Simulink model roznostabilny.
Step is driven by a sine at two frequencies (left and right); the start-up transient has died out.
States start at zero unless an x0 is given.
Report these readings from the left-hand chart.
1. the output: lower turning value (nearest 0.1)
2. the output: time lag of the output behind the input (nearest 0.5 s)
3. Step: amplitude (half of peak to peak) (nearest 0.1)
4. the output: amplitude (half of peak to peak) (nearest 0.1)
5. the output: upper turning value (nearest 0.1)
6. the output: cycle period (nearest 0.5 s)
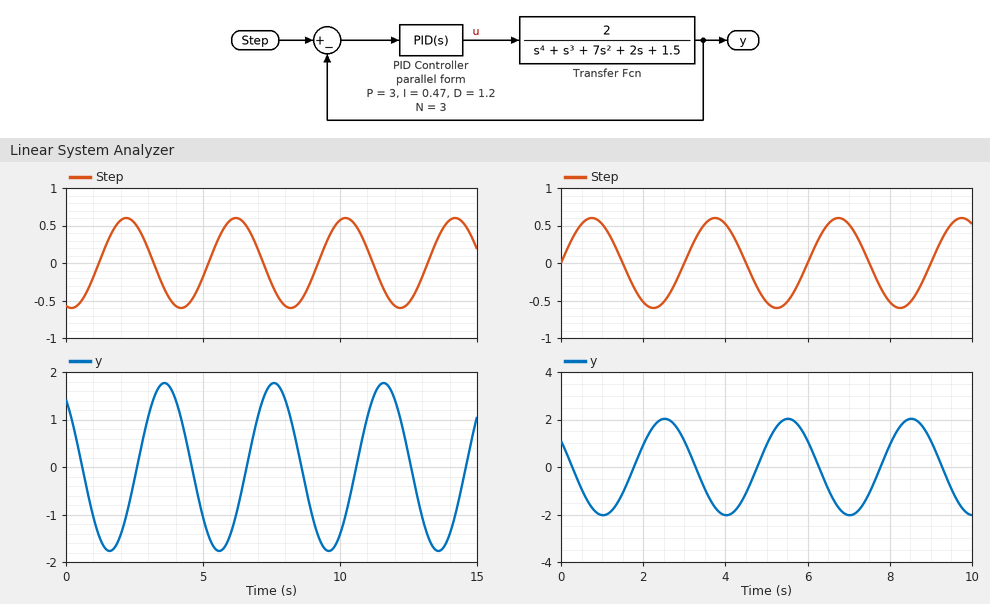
-1.8
1.5 s
0.6
1.8
1.8
4.0 s
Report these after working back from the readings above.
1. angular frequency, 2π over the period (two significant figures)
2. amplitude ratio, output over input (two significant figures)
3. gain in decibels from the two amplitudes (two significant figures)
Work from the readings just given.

1.6 rad/s
3.0
9.5 dB
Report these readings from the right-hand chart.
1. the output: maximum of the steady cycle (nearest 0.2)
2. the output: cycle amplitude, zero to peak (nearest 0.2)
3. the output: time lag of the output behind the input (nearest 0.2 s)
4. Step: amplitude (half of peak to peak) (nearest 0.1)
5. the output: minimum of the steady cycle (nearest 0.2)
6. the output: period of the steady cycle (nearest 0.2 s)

2.0
2.0
1.8 s
0.6
-2.0
3.0 s
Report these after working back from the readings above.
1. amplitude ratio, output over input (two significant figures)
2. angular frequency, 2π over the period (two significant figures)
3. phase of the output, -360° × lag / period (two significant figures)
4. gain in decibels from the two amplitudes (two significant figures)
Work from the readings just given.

3.3
2.1 rad/s
-220°
10 dB
